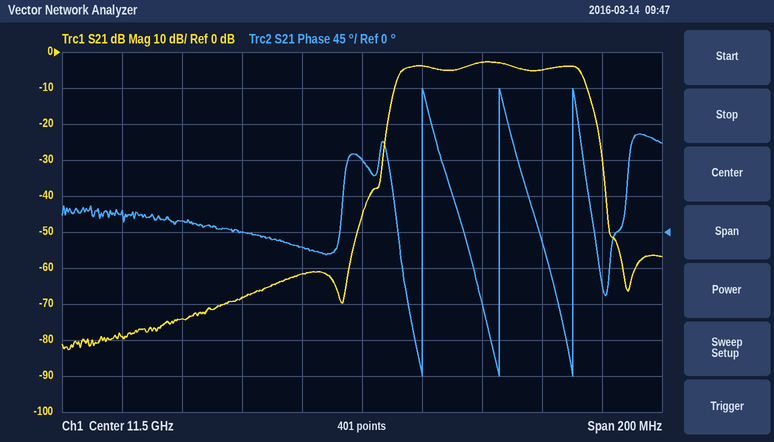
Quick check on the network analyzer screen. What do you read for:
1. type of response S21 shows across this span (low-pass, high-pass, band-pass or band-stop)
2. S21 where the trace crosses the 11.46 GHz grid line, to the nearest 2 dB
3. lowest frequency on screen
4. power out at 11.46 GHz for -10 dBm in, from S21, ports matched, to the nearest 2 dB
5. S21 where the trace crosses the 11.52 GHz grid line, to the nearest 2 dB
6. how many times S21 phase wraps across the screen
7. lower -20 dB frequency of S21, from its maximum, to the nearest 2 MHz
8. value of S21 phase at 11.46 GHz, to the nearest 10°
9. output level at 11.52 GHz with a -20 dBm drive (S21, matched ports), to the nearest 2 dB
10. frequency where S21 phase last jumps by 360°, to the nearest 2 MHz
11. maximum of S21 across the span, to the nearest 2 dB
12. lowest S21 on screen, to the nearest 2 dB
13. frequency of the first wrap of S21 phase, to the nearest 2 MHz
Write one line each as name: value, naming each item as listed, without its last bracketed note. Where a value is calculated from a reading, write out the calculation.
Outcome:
type of response S21 shows across this span: band-pass
S21 where the trace crosses the 11.46 GHz grid line, to the nearest 2 dB: -68 dB
lowest frequency on screen: 11.4 GHz
power out at 11.46 GHz for -10 dBm in, from S21, ports matched, to the nearest 2 dB: -10 dBm + (-68 dB) = -78 dBm
S21 where the trace crosses the 11.52 GHz grid line, to the nearest 2 dB: -4 dB
how many times S21 phase wraps across the screen: 3
lower -20 dB frequency of S21, from its maximum, to the nearest 2 MHz: 11.508 GHz
value of S21 phase at 11.46 GHz, to the nearest 10°: 0°
output level at 11.52 GHz with a -20 dBm drive (S21, matched ports), to the nearest 2 dB: -20 dBm + (-4 dB) = -24 dBm
frequency where S21 phase last jumps by 360°, to the nearest 2 MHz: 11.570 GHz
maximum of S21 across the span, to the nearest 2 dB: -2 dB
lowest S21 on screen, to the nearest 2 dB: -82 dB
frequency of the first wrap of S21 phase, to the nearest 2 MHz: 11.520 GHz
